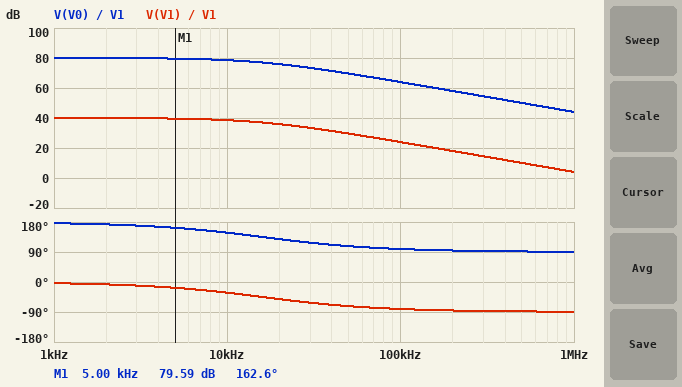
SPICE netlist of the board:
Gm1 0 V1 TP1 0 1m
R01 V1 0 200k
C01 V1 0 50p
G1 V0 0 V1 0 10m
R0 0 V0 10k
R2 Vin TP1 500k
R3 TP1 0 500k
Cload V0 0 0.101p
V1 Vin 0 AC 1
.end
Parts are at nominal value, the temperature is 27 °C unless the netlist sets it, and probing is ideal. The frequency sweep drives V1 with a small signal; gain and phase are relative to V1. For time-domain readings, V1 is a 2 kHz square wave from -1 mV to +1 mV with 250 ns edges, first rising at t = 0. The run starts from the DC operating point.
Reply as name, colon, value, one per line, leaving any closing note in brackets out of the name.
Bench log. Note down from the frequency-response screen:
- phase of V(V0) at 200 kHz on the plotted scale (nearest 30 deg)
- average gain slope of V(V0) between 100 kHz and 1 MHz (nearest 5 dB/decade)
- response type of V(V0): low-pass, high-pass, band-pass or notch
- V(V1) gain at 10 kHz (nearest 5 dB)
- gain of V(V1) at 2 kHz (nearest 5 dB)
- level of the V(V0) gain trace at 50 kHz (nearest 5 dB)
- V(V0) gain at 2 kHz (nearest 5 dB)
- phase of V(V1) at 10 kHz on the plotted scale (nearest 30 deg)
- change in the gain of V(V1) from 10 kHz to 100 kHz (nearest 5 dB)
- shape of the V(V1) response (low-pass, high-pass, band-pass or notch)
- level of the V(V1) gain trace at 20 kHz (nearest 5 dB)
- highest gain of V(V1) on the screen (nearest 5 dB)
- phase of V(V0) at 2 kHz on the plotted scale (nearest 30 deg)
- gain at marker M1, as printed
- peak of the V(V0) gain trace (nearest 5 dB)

phase of V(V0) at 200 kHz on the plotted scale: 90 deg
average gain slope of V(V0) between 100 kHz and 1 MHz: -20 dB/decade
response type of V(V0): low-pass, high-pass, band-pass or notch: low-pass
V(V1) gain at 10 kHz: 40 dB
gain of V(V1) at 2 kHz: 40 dB
level of the V(V0) gain trace at 50 kHz: 70 dB
V(V0) gain at 2 kHz: 80 dB
phase of V(V1) at 10 kHz on the plotted scale: -30 deg
change in the gain of V(V1) from 10 kHz to 100 kHz: -15 dB
shape of the V(V1) response: low-pass
level of the V(V1) gain trace at 20 kHz: 35 dB
highest gain of V(V1) on the screen: 40 dB
phase of V(V0) at 2 kHz on the plotted scale: 180 deg
gain at marker M1, as printed: 79.59 dB
peak of the V(V0) gain trace: 80 dB
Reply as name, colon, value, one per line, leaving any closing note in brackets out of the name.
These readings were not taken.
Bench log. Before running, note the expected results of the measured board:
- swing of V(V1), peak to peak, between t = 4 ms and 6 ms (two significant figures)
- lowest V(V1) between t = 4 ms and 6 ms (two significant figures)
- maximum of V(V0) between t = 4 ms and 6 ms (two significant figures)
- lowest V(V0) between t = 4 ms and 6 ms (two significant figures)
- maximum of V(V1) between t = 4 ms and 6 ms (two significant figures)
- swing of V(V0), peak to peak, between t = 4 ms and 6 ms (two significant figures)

swing of V(V1), peak to peak, between t = 4 ms and 6 ms: 200 mV
lowest V(V1) between t = 4 ms and 6 ms: -100 mV
maximum of V(V0) between t = 4 ms and 6 ms: 10 V
lowest V(V0) between t = 4 ms and 6 ms: -10 V
maximum of V(V1) between t = 4 ms and 6 ms: 100 mV
swing of V(V0), peak to peak, between t = 4 ms and 6 ms: 20 V
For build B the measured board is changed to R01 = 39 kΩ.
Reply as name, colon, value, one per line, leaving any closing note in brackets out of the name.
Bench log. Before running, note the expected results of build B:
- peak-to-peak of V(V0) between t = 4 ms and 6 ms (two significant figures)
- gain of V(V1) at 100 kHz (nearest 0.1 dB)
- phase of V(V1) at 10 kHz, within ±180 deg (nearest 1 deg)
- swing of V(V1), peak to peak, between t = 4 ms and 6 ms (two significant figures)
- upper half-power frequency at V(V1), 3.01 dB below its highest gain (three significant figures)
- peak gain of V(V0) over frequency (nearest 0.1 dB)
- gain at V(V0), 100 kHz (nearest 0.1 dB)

peak-to-peak of V(V0) between t = 4 ms and 6 ms: 3.9 V
gain of V(V1) at 100 kHz: 21.8 dB
phase of V(V1) at 10 kHz, within ±180 deg: -7 deg
swing of V(V1), peak to peak, between t = 4 ms and 6 ms: 39 mV
upper half-power frequency at V(V1), 3.01 dB below its highest gain: 81.6 kHz
peak gain of V(V0) over frequency: 65.8 dB
gain at V(V0), 100 kHz: 61.8 dB
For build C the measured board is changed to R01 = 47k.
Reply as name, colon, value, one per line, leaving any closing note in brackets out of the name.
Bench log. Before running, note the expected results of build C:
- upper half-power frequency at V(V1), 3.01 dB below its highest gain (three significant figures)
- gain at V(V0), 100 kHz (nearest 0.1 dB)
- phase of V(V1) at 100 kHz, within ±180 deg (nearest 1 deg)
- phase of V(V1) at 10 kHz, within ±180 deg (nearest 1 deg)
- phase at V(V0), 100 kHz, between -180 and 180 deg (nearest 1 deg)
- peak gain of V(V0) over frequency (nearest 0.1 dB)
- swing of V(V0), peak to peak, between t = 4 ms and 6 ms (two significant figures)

upper half-power frequency at V(V1), 3.01 dB below its highest gain: 67.7 kHz
gain at V(V0), 100 kHz: 62.4 dB
phase of V(V1) at 100 kHz, within ±180 deg: -56 deg
phase of V(V1) at 10 kHz, within ±180 deg: -8 deg
phase at V(V0), 100 kHz, between -180 and 180 deg: 124 deg
peak gain of V(V0) over frequency: 67.4 dB
swing of V(V0), peak to peak, between t = 4 ms and 6 ms: 4.7 V
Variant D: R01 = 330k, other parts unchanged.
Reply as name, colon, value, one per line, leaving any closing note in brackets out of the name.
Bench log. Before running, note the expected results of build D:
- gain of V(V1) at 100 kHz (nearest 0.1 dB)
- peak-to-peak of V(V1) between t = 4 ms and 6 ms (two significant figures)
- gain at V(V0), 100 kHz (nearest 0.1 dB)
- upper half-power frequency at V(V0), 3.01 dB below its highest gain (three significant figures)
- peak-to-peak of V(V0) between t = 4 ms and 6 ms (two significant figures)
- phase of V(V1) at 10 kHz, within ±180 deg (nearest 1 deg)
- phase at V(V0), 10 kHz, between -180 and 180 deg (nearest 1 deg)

gain of V(V1) at 100 kHz: 24.0 dB
peak-to-peak of V(V1) between t = 4 ms and 6 ms: 330 mV
gain at V(V0), 100 kHz: 64.0 dB
upper half-power frequency at V(V0), 3.01 dB below its highest gain: 9.65 kHz
peak-to-peak of V(V0) between t = 4 ms and 6 ms: 33 V
phase of V(V1) at 10 kHz, within ±180 deg: -46 deg
phase at V(V0), 10 kHz, between -180 and 180 deg: 134 deg
